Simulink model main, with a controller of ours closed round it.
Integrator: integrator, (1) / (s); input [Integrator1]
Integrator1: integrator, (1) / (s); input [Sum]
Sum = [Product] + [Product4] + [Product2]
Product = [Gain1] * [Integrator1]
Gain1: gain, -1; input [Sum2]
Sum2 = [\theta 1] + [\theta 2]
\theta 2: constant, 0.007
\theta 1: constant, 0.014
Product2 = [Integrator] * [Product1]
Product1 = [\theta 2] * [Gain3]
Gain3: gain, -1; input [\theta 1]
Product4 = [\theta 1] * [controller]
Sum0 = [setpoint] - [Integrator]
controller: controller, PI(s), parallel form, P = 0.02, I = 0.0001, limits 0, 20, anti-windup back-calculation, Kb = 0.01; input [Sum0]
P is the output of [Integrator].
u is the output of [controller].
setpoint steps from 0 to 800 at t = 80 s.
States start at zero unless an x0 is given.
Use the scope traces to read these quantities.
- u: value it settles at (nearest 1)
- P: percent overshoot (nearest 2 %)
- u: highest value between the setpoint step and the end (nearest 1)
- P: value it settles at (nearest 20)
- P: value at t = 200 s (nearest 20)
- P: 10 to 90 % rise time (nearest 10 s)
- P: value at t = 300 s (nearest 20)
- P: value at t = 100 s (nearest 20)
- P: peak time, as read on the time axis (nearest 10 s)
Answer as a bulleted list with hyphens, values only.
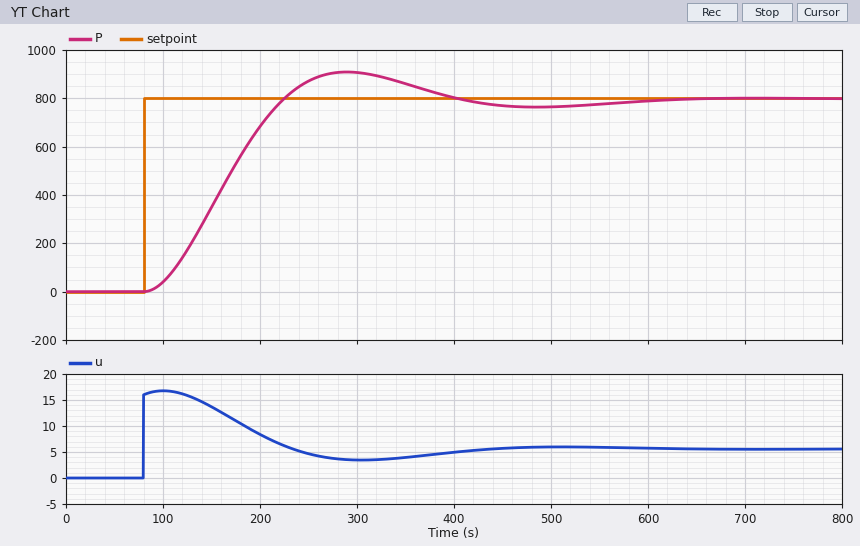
- 6
- 14 %
- 17
- 800
- 680
- 100 s
- 900
- 40
- 290 s
